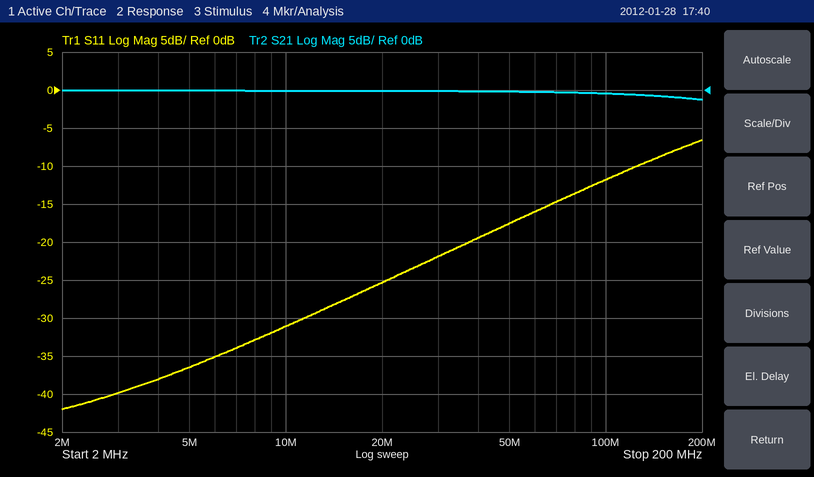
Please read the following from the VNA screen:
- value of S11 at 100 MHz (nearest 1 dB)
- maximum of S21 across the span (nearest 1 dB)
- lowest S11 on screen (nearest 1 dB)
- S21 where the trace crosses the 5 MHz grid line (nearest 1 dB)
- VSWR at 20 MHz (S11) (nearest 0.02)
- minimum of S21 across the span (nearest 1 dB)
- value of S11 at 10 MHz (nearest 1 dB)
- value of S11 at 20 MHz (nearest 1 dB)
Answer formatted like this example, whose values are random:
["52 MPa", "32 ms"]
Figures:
["-12 dB", "0 dB", "-42 dB", "0 dB", "1.12", "-1 dB", "-31 dB", "-25 dB"]
